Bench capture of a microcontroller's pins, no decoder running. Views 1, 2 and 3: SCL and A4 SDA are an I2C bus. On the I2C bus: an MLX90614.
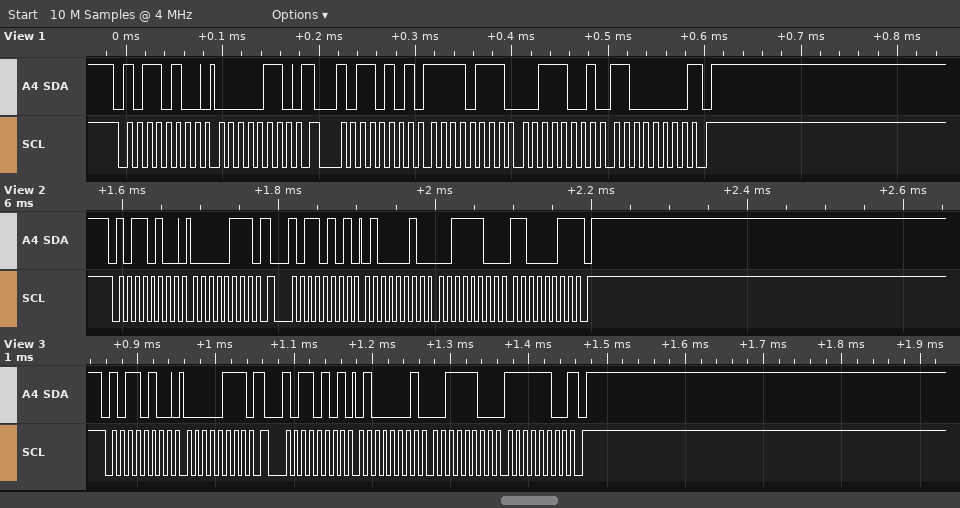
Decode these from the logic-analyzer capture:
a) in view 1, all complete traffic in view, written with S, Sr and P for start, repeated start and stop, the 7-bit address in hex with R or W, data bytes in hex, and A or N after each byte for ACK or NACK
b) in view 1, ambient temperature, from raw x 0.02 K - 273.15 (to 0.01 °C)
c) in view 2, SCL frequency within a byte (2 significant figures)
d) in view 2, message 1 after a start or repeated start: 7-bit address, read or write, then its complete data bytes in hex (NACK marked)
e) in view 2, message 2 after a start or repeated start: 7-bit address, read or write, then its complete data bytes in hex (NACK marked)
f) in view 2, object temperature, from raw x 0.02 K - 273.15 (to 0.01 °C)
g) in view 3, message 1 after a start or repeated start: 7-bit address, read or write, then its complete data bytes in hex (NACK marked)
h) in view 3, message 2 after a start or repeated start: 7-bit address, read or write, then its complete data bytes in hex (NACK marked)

S 5AW A 06 A Sr 5AR A F7 A 39 A C0 N P
23.63 °C
100 kHz
0x5A write: 07
0x5A read: 42 3C C3 NACK
35.37 °C
0x5A write: 07
0x5A read: 41 3C FC NACK
